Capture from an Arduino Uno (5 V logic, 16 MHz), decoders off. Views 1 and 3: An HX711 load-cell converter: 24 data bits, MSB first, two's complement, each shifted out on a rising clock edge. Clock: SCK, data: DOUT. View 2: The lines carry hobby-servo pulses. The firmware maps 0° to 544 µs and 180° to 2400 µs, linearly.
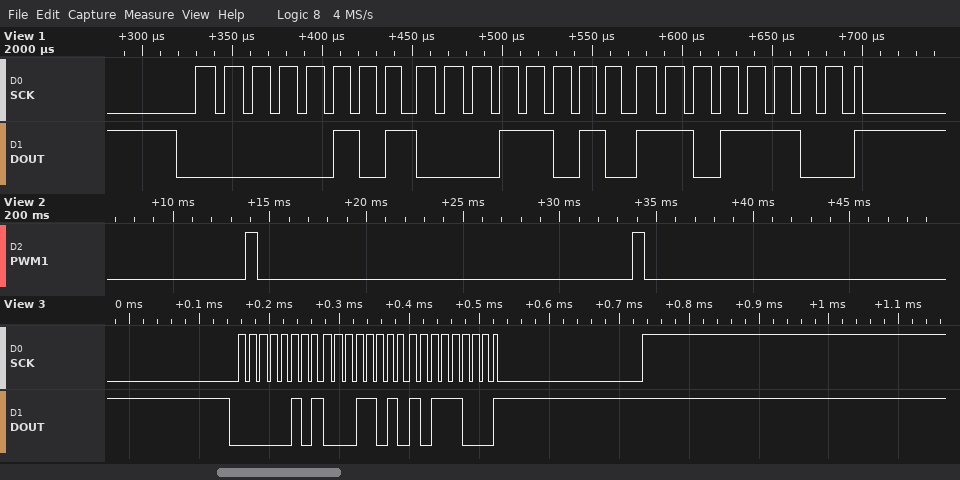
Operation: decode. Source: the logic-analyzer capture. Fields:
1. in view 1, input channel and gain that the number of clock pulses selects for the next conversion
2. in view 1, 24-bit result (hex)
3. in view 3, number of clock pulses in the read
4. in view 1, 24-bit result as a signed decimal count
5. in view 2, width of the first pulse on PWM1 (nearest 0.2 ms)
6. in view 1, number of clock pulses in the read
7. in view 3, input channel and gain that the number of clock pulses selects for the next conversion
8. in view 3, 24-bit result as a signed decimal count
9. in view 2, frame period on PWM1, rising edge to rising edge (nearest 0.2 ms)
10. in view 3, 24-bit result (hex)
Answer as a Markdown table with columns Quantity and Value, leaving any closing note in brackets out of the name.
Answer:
| Quantity | Value |
|---|---|
| in view 1, input channel and gain that the number of clock pulses selects for the next conversion | channel A, gain 128 |
| in view 1, 24-bit result | 0x051ADC |
| in view 3, number of clock pulses in the read | 26 |
| in view 1, 24-bit result as a signed decimal count | 334556 |
| in view 2, width of the first pulse on PWM1 | 0.6 ms |
| in view 1, number of clock pulses in the read | 25 |
| in view 3, input channel and gain that the number of clock pulses selects for the next conversion | channel B, gain 32 |
| in view 3, 24-bit result as a signed decimal count | 334520 |
| in view 2, frame period on PWM1, rising edge to rising edge | 20.0 ms |
| in view 3, 24-bit result | 0x051AB8 |
